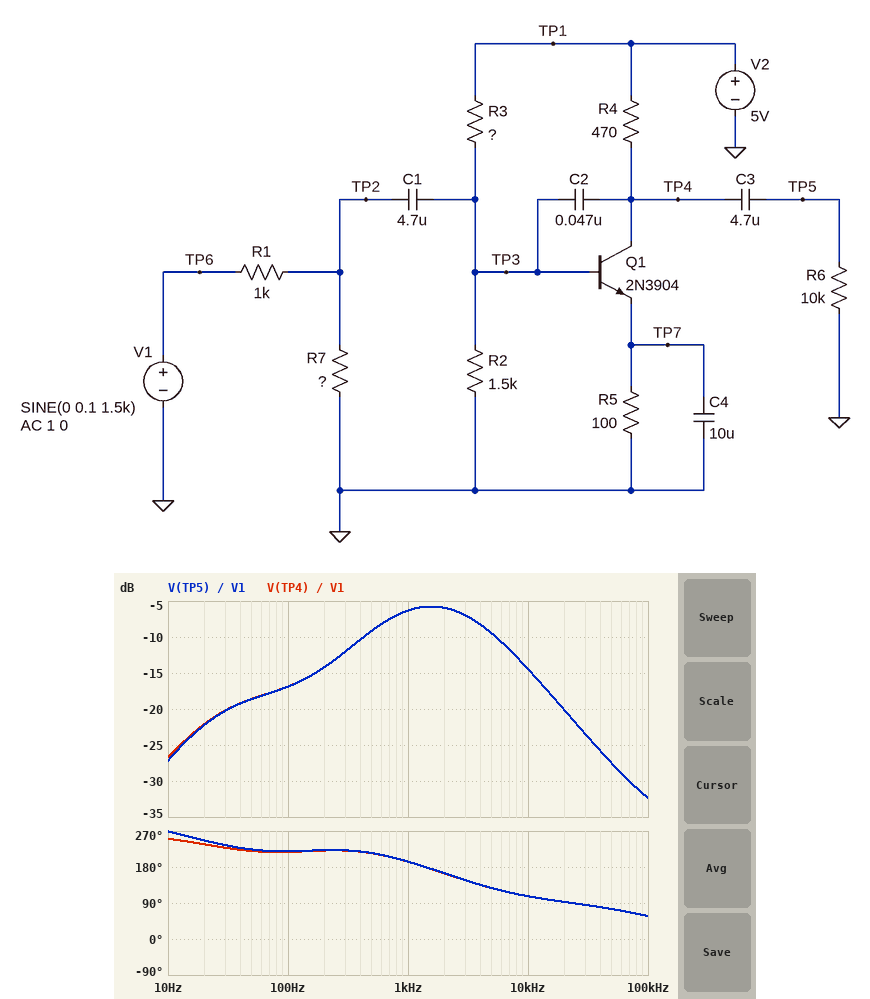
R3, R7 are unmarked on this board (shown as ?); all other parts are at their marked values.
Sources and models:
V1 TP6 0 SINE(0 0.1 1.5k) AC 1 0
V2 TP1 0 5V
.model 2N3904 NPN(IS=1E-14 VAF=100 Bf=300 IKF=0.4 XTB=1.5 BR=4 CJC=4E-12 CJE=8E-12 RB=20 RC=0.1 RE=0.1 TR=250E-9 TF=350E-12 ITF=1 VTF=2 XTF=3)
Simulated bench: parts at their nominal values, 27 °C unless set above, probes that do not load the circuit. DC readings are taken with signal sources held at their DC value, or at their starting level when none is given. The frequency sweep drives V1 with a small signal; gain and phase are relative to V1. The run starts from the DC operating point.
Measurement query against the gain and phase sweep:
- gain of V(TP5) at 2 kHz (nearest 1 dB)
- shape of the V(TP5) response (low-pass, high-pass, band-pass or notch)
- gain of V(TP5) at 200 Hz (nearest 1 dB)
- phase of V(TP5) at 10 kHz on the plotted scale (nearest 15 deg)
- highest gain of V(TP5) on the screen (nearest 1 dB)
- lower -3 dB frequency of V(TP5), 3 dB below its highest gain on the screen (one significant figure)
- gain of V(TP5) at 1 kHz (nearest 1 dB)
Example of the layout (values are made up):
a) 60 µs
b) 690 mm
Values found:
a) -6 dB
b) band-pass
c) -14 dB
d) 105 deg
e) -6 dB
f) 500 Hz
g) -6 dB
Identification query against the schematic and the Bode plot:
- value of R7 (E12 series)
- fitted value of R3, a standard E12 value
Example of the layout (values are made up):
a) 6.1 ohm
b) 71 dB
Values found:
a) 39 Ω
b) 8.2 kΩ
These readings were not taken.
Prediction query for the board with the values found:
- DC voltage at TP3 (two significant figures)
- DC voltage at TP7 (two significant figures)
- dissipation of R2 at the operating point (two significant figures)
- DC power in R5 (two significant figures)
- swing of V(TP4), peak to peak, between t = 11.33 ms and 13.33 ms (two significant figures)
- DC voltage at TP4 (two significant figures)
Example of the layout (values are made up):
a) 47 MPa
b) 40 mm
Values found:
a) 770 mV
b) 110 mV
c) 390 µW
d) 120 µW
e) 100 mV
f) 4.5 V
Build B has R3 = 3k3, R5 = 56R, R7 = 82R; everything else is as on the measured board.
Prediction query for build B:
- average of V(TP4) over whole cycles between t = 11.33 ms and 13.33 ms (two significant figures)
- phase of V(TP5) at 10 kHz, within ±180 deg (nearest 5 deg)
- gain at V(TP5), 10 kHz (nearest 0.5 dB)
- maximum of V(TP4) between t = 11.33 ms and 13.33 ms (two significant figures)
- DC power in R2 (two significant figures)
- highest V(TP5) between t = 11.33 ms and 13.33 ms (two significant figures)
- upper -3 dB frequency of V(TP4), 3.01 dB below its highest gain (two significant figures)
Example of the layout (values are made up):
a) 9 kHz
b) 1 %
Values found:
a) 600 mV
b) 165 deg
c) -25.0 dB
d) 610 mV
e) 1.1 mW
f) 6.2 mV
g) 35 kHz
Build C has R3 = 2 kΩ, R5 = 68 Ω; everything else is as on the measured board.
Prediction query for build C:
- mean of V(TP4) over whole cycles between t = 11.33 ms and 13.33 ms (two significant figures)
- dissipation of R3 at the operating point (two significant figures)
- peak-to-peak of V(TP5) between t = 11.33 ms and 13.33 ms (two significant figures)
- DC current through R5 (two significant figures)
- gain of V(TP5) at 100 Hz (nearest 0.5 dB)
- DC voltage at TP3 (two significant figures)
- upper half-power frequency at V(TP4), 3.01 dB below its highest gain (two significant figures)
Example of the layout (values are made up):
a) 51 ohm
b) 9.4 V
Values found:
a) 720 mV
b) 6.4 mW
c) 2.1 mV
d) 10 mA
e) -49.0 dB
f) 1.4 V
g) 86 kHz
